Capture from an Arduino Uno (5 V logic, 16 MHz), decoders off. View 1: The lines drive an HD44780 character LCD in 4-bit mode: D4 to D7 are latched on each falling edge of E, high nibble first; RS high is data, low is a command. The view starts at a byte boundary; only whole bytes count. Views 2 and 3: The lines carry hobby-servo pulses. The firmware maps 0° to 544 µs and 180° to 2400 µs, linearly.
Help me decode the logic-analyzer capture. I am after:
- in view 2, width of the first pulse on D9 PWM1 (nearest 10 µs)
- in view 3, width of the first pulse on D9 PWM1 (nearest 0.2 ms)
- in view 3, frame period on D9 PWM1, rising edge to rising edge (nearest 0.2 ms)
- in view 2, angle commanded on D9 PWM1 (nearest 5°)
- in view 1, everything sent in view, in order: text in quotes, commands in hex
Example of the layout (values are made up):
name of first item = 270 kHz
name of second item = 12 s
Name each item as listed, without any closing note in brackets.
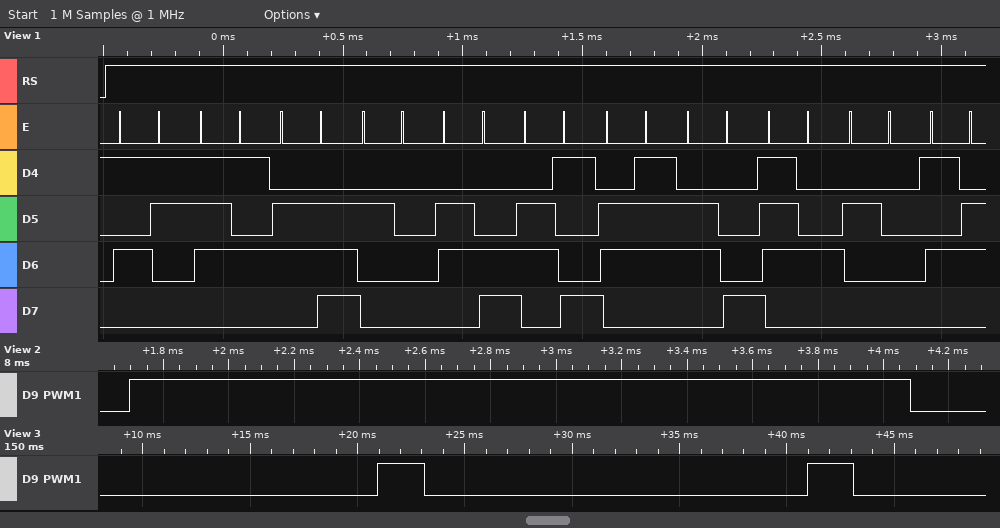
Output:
in view 2, width of the first pulse on D9 PWM1 = 2390 µs
in view 3, width of the first pulse on D9 PWM1 = 2.2 ms
in view 3, frame period on D9 PWM1, rising edge to rising edge = 20.0 ms
in view 2, angle commanded on D9 PWM1 = 180°
in view 1, everything sent in view, in order: text in quotes, commands in hex = "Sun light V"
